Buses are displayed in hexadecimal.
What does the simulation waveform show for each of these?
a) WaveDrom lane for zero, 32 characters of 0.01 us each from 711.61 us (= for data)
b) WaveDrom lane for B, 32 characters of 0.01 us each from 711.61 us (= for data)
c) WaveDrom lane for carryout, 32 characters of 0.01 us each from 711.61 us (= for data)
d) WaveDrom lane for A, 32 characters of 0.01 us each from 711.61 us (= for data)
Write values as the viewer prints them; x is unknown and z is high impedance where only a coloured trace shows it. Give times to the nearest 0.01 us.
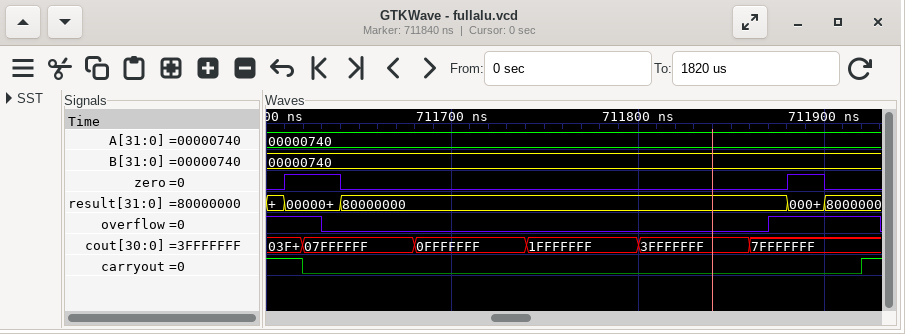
{name: 'zero', wave: '1..0.......................1.0..'}
{name: 'B', wave: '=...............................', data: '00000740'}
{name: 'carryout', wave: '10.............................1'}
{name: 'A', wave: '=...............................', data: '00000740'}
